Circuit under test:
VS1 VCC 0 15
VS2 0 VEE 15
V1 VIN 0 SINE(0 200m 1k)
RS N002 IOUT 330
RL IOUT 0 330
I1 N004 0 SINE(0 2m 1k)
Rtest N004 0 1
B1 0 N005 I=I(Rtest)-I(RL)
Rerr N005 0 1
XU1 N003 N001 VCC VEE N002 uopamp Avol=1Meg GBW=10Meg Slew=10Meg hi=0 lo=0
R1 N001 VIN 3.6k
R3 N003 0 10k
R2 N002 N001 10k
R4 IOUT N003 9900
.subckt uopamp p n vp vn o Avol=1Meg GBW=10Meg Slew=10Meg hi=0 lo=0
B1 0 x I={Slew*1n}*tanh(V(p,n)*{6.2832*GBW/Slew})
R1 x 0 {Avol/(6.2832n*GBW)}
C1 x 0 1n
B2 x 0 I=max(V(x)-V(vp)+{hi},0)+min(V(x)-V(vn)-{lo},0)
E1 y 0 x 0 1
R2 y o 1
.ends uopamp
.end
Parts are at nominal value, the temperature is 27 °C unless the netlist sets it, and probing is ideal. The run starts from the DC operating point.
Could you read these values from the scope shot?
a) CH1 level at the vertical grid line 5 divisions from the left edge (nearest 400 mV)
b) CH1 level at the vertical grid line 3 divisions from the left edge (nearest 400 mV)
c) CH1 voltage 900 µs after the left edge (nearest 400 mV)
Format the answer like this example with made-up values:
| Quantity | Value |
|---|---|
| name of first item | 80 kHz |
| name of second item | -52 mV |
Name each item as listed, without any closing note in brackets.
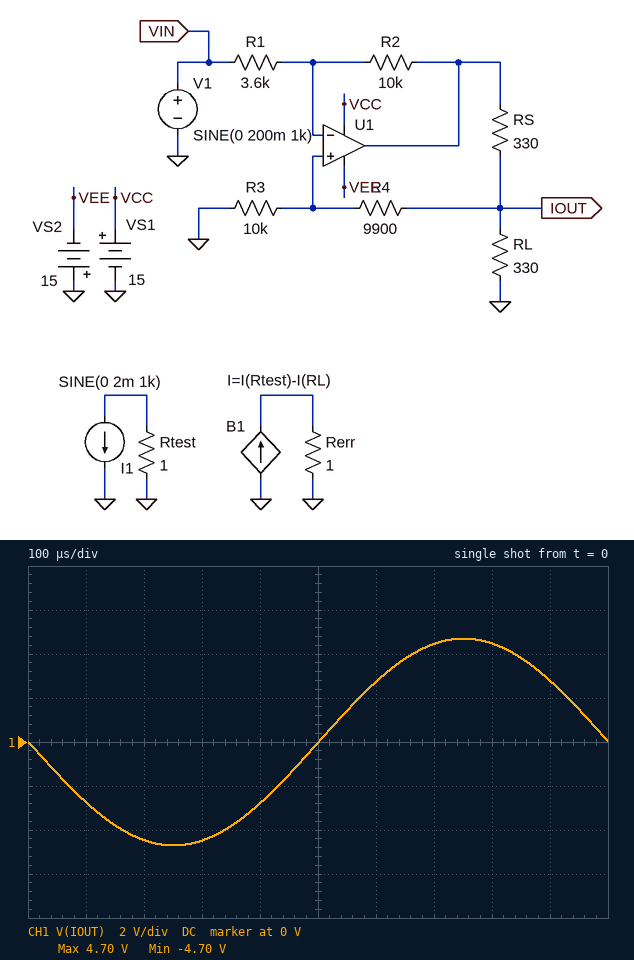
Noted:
| Quantity | Value |
|---|---|
| CH1 level at the vertical grid line 5 divisions from the left edge | 0 V |
| CH1 level at the vertical grid line 3 divisions from the left edge | -4.4 V |
| CH1 voltage 900 µs after the left edge | 2.8 V |
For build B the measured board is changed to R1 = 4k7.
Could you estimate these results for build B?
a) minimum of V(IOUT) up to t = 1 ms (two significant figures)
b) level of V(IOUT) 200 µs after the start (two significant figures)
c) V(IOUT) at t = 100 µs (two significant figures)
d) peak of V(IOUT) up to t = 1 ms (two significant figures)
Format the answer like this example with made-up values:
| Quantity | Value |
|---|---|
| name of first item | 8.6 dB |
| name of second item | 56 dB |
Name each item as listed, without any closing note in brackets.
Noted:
| Quantity | Value |
|---|---|
| minimum of V(IOUT) up to t = 1 ms | -960 mV |
| level of V(IOUT) 200 µs after the start | -910 mV |
| V(IOUT) at t = 100 µs | -560 mV |
| peak of V(IOUT) up to t = 1 ms | 960 mV |
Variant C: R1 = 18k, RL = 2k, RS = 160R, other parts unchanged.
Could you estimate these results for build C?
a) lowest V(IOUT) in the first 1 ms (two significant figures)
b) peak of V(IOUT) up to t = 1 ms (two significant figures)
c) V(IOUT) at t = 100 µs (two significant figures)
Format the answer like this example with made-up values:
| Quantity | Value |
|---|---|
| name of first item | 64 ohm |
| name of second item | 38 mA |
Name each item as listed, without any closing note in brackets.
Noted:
| Quantity | Value |
|---|---|
| lowest V(IOUT) in the first 1 ms | -360 mV |
| peak of V(IOUT) up to t = 1 ms | 360 mV |
| V(IOUT) at t = 100 µs | -210 mV |
